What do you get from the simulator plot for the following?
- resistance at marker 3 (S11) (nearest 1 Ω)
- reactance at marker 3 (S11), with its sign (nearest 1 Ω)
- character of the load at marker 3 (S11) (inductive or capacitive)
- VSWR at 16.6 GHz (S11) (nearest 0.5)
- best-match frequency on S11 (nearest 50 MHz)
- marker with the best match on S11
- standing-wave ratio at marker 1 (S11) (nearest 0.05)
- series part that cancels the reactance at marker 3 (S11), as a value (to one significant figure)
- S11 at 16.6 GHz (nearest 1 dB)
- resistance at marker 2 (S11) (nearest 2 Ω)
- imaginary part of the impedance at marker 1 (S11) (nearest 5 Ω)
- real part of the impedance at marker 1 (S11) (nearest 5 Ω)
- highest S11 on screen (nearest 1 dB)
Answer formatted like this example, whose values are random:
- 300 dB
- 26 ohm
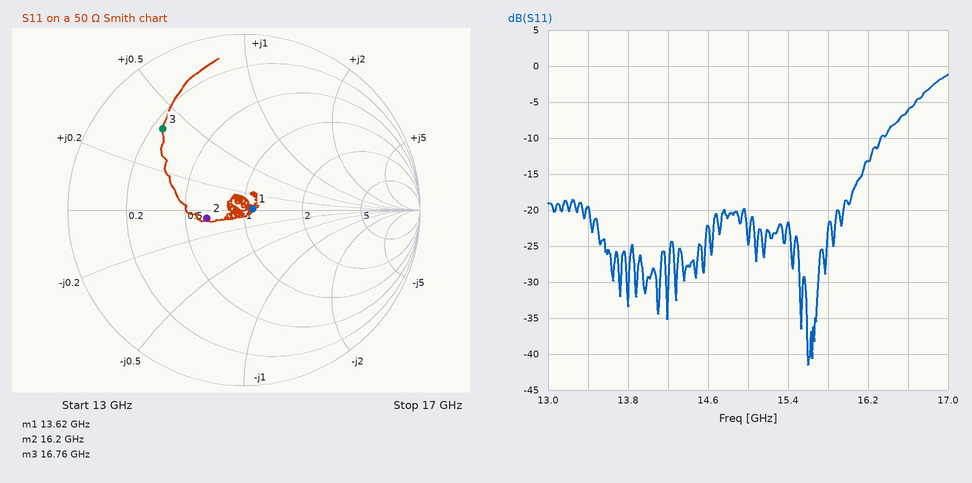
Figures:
- 12 Ω
- +20 Ω
- inductive
- 3.0
- 15.60 GHz
- marker 1
- 1.10
- 500 fF
- -6 dB
- 32 Ω
- 0 Ω
- 55 Ω
- -1 dB
